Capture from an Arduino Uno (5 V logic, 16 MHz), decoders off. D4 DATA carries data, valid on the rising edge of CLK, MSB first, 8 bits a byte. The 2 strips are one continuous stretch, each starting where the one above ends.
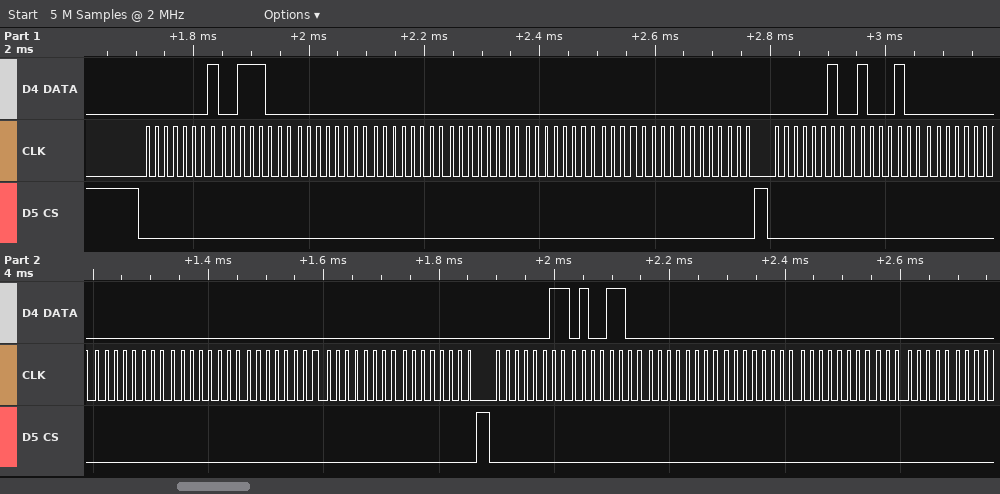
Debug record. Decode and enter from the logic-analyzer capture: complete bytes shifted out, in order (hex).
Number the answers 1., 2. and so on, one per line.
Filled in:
1. 01 38 00 00 00 00 00 00 02 44 00 00 00 00 00 00 03 4C 00 00 00 00
